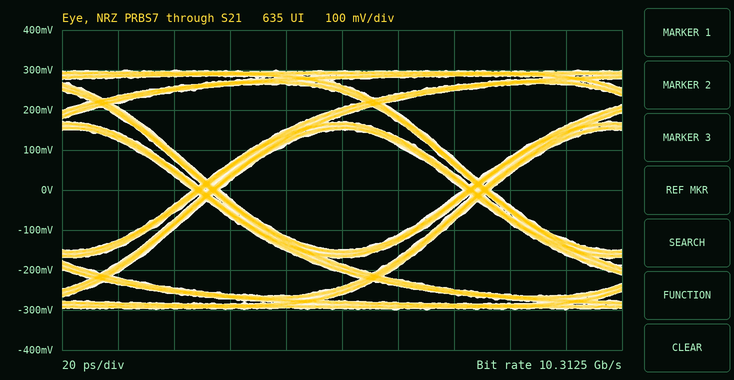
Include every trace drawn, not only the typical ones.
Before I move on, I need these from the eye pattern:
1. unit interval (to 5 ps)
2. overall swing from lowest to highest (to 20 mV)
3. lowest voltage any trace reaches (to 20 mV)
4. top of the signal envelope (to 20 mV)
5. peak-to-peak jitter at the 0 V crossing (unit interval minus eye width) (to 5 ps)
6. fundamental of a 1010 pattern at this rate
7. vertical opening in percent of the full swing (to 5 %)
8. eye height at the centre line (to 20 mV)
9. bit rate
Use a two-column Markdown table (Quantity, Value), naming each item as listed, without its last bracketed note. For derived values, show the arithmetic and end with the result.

| Quantity | Value |
|---|---|
| unit interval | 95 ps |
| overall swing from lowest to highest | 600 mV |
| lowest voltage any trace reaches | -300 mV |
| top of the signal envelope | 300 mV |
| peak-to-peak jitter at the 0 V crossing (unit interval minus eye width) | 10 ps |
| fundamental of a 1010 pattern at this rate | 5.15625 GHz |
| vertical opening in percent of the full swing | 300 mV / 600 mV ≈ 50 % |
| eye height at the centre line | 300 mV |
| bit rate | 10.3125 Gb/s |
